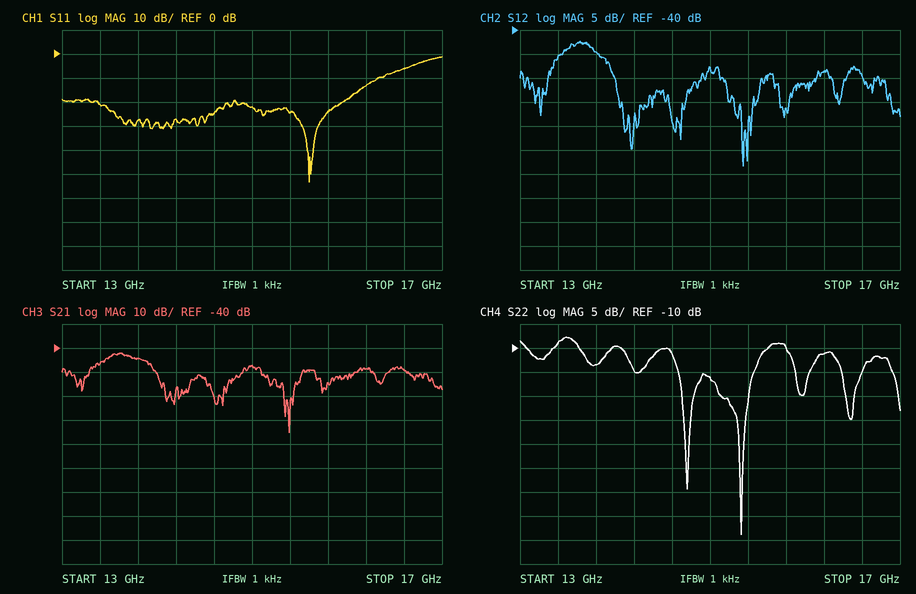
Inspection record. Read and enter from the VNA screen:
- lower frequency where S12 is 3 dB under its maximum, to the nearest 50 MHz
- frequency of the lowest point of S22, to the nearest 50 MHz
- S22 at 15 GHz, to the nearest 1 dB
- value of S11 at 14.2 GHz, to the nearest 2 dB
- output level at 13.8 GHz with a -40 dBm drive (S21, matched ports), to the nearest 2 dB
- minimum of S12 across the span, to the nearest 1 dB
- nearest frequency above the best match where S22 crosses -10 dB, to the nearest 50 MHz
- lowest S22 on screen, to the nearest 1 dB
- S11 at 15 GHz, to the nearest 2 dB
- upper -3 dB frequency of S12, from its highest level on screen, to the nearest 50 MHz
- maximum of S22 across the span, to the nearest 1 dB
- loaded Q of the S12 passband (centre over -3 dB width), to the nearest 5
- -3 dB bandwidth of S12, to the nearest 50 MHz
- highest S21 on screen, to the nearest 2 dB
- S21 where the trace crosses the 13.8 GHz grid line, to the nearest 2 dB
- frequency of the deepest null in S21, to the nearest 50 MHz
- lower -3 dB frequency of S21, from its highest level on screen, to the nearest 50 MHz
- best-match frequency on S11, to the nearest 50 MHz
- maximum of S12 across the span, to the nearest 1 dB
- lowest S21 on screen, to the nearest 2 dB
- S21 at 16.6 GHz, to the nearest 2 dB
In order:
13.40 GHz
15.35 GHz
-16 dB
-28 dB
-84 dBm
-68 dB
15.60 GHz
-49 dB
-22 dB
13.85 GHz
-8 dB
30
450 MHz
-42 dB
-44 dB
15.40 GHz
13.45 GHz
15.60 GHz
-42 dB
-76 dB
-50 dB
